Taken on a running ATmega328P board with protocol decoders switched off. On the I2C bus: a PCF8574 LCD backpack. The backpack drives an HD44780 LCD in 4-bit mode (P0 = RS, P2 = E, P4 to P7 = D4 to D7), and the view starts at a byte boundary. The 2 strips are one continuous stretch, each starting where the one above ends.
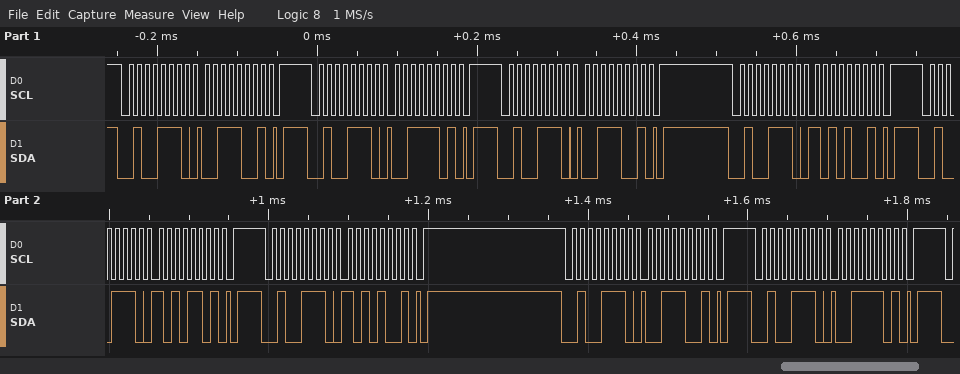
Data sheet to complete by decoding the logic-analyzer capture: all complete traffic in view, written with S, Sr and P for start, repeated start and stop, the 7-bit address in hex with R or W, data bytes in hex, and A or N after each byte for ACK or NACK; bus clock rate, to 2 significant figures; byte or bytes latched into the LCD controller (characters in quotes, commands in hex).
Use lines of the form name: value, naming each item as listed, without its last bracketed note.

all complete traffic in view, written with S, Sr and P for start, repeated start and stop, the 7-bit address in hex with R or W, data bytes in hex, and A or N after each byte for ACK or NACK: S 27W A 39 A P S 27W A 3D A P S 27W A 39 A P S 27W A A9 A P S 27W A AD A P S 27W A A9 A P S 27W A 39 A P S 27W A 3D A P
bus clock rate, to 2 significant figures: 100 kHz
byte or bytes latched into the LCD controller: ':'
